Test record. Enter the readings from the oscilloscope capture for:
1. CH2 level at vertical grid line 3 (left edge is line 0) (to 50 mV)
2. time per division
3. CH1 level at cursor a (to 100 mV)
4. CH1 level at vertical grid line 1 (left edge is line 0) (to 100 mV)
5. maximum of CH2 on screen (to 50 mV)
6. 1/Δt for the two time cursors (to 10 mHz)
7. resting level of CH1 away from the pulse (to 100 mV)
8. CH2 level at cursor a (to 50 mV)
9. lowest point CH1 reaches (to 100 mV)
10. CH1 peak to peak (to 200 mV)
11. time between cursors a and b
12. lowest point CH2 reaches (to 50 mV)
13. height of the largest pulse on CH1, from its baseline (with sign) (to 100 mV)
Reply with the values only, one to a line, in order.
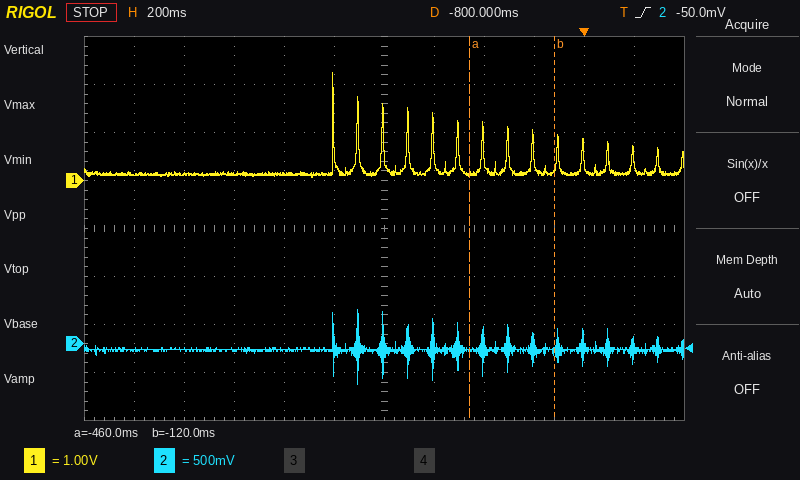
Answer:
-50 mV
200 ms
100 mV
100 mV
350 mV
2.94 Hz
100 mV
-50 mV
100 mV
2.2 V
340 ms
-400 mV
+2.1 V
